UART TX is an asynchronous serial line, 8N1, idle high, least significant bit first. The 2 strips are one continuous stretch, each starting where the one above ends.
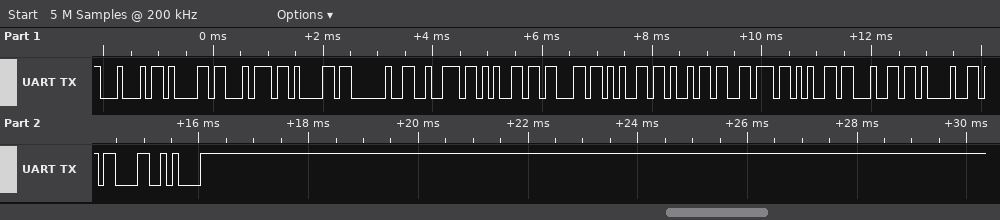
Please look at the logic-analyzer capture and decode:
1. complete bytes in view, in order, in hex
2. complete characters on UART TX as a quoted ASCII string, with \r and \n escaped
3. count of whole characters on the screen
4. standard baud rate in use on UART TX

44 61 74 61 20 72 65 63 65 69 76 65 64 21 0D 0A
"Data received!\r\n"
16
9600 baud
